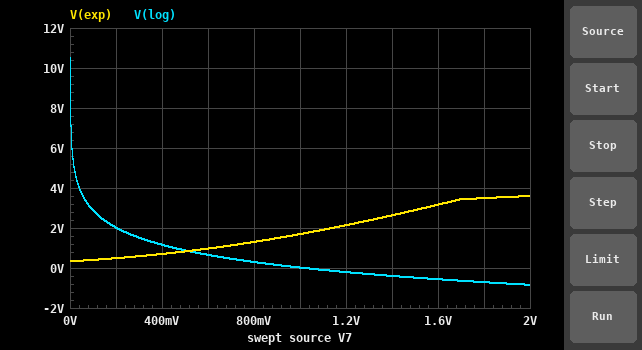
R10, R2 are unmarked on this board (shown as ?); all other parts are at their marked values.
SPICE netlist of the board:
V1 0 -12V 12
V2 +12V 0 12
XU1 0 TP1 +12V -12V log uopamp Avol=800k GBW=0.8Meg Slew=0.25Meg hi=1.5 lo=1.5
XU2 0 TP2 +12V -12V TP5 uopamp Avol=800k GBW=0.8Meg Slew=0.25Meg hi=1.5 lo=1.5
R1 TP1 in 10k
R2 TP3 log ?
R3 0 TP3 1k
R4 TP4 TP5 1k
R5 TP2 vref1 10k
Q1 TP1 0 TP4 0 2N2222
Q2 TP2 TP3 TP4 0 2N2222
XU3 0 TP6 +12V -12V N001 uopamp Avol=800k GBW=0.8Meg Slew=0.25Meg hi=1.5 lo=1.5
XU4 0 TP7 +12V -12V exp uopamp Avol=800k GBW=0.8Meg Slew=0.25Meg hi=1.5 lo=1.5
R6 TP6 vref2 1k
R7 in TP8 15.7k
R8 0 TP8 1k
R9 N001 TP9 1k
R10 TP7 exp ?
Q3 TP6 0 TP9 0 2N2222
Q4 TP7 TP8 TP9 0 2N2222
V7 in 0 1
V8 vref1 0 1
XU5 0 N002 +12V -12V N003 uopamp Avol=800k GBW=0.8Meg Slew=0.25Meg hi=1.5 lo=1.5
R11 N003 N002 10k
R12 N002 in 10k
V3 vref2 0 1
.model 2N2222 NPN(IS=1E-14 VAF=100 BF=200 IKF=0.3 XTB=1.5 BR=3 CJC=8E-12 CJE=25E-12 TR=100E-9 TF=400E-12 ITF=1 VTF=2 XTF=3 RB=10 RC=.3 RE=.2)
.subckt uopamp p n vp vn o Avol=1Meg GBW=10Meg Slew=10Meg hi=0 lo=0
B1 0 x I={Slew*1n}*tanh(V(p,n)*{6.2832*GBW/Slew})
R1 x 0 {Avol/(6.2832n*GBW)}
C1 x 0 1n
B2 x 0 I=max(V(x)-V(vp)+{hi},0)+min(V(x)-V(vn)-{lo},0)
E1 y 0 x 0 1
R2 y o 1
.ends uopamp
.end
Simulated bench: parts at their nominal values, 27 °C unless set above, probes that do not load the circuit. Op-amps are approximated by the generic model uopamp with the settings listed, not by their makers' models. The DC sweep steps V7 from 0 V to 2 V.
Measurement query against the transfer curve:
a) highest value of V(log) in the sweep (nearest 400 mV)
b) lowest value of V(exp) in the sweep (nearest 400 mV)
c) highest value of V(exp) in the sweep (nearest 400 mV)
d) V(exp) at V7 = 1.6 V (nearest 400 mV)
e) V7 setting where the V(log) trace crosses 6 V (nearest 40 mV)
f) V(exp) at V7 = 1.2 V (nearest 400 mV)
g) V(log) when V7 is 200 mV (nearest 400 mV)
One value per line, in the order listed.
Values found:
10.4 V
400 mV
3.6 V
3.2 V
0 V
2.0 V
2.0 V
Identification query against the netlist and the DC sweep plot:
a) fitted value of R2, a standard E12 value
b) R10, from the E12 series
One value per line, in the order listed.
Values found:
47 kΩ
390 Ω
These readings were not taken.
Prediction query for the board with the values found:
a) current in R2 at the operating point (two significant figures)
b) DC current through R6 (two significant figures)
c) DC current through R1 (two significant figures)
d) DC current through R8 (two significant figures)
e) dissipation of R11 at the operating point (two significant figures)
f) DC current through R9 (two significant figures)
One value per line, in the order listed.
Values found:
500 nA
1.0 mA
100 µA
39 µA
100 µW
5.4 mA
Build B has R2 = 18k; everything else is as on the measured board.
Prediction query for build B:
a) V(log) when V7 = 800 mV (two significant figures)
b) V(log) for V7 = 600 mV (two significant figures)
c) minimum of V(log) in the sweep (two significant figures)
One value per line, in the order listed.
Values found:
120 mV
260 mV
-330 mV
